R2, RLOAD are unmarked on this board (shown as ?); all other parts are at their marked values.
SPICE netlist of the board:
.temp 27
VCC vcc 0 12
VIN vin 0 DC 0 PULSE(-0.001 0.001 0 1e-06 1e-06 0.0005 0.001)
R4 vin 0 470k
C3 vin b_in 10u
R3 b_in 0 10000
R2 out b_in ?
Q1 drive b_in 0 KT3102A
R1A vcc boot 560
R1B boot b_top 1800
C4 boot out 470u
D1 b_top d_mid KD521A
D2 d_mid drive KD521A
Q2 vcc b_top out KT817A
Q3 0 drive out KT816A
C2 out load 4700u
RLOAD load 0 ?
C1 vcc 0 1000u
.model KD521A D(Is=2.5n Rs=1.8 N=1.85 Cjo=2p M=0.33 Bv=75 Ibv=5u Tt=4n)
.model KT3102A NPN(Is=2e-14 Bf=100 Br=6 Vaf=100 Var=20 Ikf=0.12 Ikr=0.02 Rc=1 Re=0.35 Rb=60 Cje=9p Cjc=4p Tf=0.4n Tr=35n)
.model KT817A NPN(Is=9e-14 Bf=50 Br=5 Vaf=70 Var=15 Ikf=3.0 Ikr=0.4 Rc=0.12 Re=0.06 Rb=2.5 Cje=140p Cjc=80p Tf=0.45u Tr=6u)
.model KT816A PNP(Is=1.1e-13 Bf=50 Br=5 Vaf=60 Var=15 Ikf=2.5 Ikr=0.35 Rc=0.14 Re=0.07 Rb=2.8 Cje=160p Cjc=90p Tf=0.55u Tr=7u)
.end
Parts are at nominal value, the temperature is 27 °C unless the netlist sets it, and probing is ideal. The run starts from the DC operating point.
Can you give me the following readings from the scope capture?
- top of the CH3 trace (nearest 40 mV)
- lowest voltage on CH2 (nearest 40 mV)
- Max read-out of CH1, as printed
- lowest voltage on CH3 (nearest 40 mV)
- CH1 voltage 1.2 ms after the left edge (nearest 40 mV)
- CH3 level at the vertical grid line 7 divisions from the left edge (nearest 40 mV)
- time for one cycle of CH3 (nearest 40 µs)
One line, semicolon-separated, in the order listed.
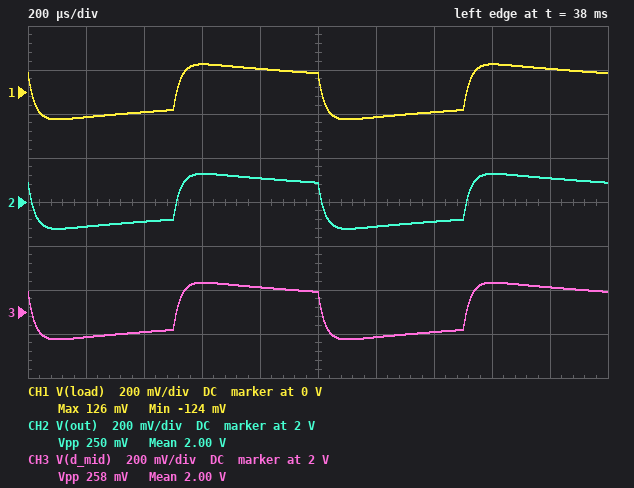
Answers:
2.12 V; 1.88 V; 126 mV; 1.88 V; -120 mV; 1.92 V; 1.00 ms
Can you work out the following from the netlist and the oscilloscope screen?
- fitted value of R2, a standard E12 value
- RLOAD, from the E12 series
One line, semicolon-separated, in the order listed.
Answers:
12 kΩ; 18 Ω
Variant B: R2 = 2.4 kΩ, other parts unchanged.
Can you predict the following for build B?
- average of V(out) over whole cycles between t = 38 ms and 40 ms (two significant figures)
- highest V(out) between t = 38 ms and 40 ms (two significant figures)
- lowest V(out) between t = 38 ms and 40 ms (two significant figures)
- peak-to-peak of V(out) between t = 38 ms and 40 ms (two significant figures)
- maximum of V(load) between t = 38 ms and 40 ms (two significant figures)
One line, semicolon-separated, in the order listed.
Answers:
960 mV; 1.1 V; 830 mV; 300 mV; 170 mV
